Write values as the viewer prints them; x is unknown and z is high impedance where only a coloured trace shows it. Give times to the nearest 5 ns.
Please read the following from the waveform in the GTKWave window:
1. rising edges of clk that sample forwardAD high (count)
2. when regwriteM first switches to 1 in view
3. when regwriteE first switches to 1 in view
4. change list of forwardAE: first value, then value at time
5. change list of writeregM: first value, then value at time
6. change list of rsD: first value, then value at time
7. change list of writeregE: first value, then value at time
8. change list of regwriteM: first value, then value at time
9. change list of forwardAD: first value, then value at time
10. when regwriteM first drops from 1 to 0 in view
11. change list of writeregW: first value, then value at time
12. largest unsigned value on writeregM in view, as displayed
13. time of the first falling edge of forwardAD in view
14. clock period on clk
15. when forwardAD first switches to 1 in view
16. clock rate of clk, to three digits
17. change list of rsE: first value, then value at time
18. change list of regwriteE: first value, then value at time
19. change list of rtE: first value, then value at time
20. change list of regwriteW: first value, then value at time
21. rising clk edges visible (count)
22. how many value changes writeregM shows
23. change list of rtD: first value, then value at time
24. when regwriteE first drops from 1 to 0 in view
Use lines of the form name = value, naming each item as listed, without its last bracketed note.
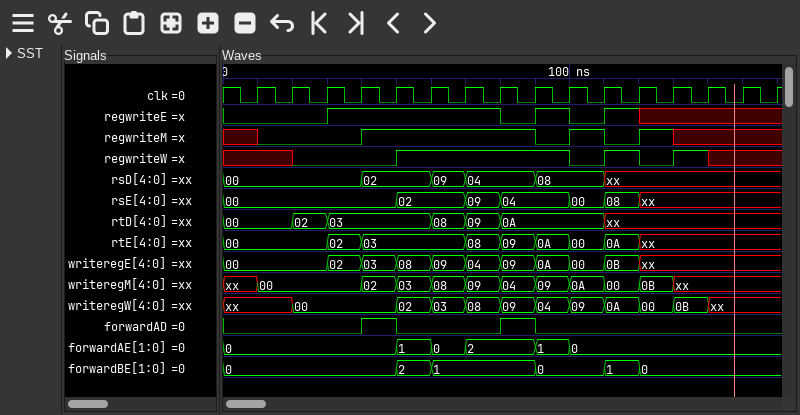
rising edges of clk that sample forwardAD high = 2
when regwriteM first switches to 1 in view = 40 ns
when regwriteE first switches to 1 in view = 30 ns
change list of forwardAE: first value, then value at time = 0, 1 at 50 ns, 0 at 60 ns, 2 at 70 ns, 1 at 90 ns, 0 at 100 ns
change list of writeregM: first value, then value at time = xx, 00 at 10 ns, 02 at 40 ns, 03 at 50 ns, 08 at 60 ns, 09 at 70 ns, 04 at 80 ns, 09 at 90 ns, 0A at 100 ns, 00 at 110 ns, 0B at 120 ns, xx at 130 ns
change list of rsD: first value, then value at time = 00, 02 at 40 ns, 09 at 60 ns, 04 at 70 ns, 08 at 90 ns, xx at 110 ns
change list of writeregE: first value, then value at time = 00, 02 at 30 ns, 03 at 40 ns, 08 at 50 ns, 09 at 60 ns, 04 at 70 ns, 09 at 80 ns, 0A at 90 ns, 00 at 100 ns, 0B at 110 ns, xx at 120 ns
change list of regwriteM: first value, then value at time = x, 0 at 10 ns, 1 at 40 ns, 0 at 90 ns, 1 at 100 ns, 0 at 110 ns, 1 at 120 ns, x at 130 ns
change list of forwardAD: first value, then value at time = 0, 1 at 40 ns, 0 at 50 ns, 1 at 80 ns, 0 at 90 ns
when regwriteM first drops from 1 to 0 in view = 90 ns
change list of writeregW: first value, then value at time = xx, 00 at 20 ns, 02 at 50 ns, 03 at 60 ns, 08 at 70 ns, 09 at 80 ns, 04 at 90 ns, 09 at 100 ns, 0A at 110 ns, 00 at 120 ns, 0B at 130 ns, xx at 140 ns
largest unsigned value on writeregM in view, as displayed = 0B
time of the first falling edge of forwardAD in view = 50 ns
clock period on clk = 10 ns
when forwardAD first switches to 1 in view = 40 ns
clock rate of clk, to three digits = 100 MHz
change list of rsE: first value, then value at time = 00, 02 at 50 ns, 09 at 70 ns, 04 at 80 ns, 00 at 100 ns, 08 at 110 ns, xx at 120 ns
change list of regwriteE: first value, then value at time = 0, 1 at 30 ns, 0 at 80 ns, 1 at 90 ns, 0 at 100 ns, 1 at 110 ns, x at 120 ns
change list of rtE: first value, then value at time = 00, 02 at 30 ns, 03 at 40 ns, 08 at 70 ns, 09 at 80 ns, 0A at 90 ns, 00 at 100 ns, 0A at 110 ns, xx at 120 ns
change list of regwriteW: first value, then value at time = x, 0 at 20 ns, 1 at 50 ns, 0 at 100 ns, 1 at 110 ns, 0 at 120 ns, 1 at 130 ns, x at 140 ns
rising clk edges visible = 16
how many value changes writeregM shows = 11
change list of rtD: first value, then value at time = 00, 02 at 20 ns, 03 at 30 ns, 08 at 60 ns, 09 at 70 ns, 0A at 80 ns, xx at 110 ns
when regwriteE first drops from 1 to 0 in view = 80 ns
